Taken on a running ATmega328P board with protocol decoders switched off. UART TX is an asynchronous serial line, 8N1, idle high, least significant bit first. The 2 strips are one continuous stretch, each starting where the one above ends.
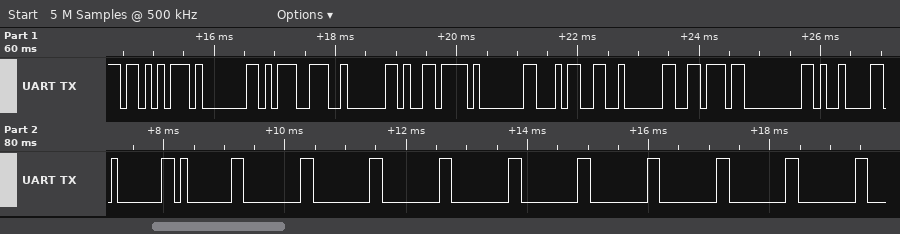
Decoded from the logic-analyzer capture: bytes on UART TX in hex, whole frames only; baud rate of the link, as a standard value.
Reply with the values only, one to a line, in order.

0xAB 0x01 0x9D 0x02 0xD9 0x01 0x34 0x02 0x76 0x00 0x09 0x01 0x01 0x00 0x00 0x00 0x00 0x00 0x00 0x00 0x00 0x00
9600 baud
